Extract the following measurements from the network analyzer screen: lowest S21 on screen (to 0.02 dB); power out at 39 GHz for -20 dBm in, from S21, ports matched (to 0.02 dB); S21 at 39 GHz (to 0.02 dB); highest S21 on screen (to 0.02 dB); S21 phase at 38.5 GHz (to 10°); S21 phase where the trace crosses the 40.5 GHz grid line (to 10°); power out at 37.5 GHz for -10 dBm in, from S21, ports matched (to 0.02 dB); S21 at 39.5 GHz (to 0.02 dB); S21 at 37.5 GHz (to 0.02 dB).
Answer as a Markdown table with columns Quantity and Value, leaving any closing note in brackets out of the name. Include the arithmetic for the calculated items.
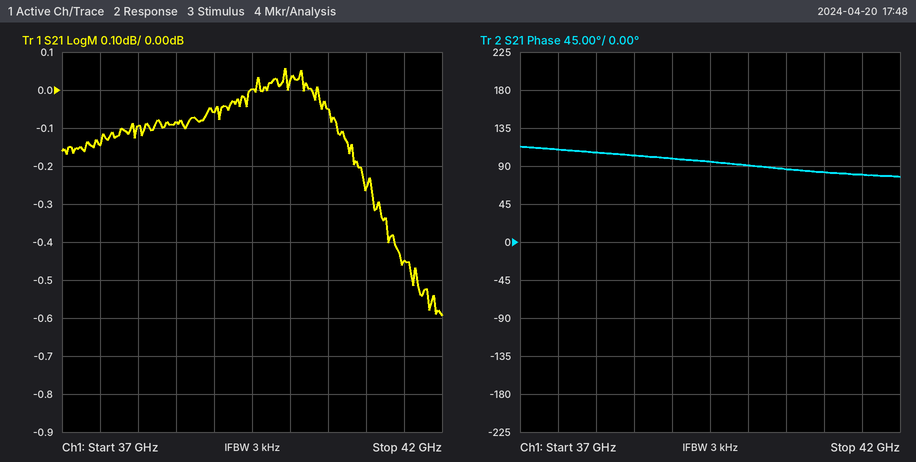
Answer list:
| Quantity | Value |
|---|---|
| lowest S21 on screen | -0.60 dB |
| power out at 39 GHz for -20 dBm in, from S21, ports matched | -20 dBm + (-0.06 dB) = -20.06 dBm |
| S21 at 39 GHz | -0.06 dB |
| highest S21 on screen | 0.06 dB |
| S21 phase at 38.5 GHz | 100° |
| S21 phase where the trace crosses the 40.5 GHz grid line | 90° |
| power out at 37.5 GHz for -10 dBm in, from S21, ports matched | -10 dBm + (-0.14 dB) = -10.14 dBm |
| S21 at 39.5 GHz | 0.00 dB |
| S21 at 37.5 GHz | -0.14 dB |
